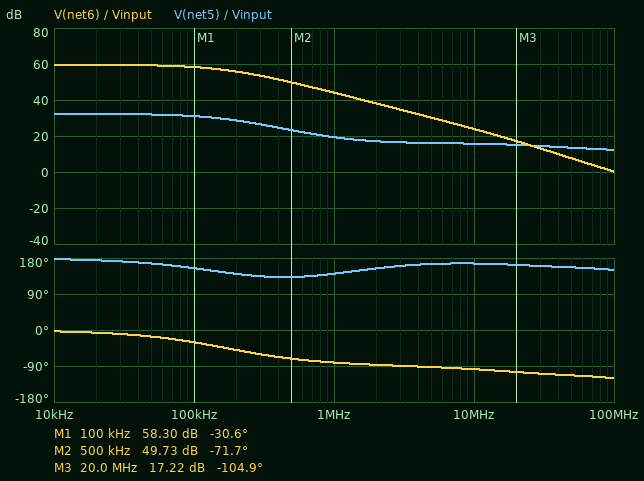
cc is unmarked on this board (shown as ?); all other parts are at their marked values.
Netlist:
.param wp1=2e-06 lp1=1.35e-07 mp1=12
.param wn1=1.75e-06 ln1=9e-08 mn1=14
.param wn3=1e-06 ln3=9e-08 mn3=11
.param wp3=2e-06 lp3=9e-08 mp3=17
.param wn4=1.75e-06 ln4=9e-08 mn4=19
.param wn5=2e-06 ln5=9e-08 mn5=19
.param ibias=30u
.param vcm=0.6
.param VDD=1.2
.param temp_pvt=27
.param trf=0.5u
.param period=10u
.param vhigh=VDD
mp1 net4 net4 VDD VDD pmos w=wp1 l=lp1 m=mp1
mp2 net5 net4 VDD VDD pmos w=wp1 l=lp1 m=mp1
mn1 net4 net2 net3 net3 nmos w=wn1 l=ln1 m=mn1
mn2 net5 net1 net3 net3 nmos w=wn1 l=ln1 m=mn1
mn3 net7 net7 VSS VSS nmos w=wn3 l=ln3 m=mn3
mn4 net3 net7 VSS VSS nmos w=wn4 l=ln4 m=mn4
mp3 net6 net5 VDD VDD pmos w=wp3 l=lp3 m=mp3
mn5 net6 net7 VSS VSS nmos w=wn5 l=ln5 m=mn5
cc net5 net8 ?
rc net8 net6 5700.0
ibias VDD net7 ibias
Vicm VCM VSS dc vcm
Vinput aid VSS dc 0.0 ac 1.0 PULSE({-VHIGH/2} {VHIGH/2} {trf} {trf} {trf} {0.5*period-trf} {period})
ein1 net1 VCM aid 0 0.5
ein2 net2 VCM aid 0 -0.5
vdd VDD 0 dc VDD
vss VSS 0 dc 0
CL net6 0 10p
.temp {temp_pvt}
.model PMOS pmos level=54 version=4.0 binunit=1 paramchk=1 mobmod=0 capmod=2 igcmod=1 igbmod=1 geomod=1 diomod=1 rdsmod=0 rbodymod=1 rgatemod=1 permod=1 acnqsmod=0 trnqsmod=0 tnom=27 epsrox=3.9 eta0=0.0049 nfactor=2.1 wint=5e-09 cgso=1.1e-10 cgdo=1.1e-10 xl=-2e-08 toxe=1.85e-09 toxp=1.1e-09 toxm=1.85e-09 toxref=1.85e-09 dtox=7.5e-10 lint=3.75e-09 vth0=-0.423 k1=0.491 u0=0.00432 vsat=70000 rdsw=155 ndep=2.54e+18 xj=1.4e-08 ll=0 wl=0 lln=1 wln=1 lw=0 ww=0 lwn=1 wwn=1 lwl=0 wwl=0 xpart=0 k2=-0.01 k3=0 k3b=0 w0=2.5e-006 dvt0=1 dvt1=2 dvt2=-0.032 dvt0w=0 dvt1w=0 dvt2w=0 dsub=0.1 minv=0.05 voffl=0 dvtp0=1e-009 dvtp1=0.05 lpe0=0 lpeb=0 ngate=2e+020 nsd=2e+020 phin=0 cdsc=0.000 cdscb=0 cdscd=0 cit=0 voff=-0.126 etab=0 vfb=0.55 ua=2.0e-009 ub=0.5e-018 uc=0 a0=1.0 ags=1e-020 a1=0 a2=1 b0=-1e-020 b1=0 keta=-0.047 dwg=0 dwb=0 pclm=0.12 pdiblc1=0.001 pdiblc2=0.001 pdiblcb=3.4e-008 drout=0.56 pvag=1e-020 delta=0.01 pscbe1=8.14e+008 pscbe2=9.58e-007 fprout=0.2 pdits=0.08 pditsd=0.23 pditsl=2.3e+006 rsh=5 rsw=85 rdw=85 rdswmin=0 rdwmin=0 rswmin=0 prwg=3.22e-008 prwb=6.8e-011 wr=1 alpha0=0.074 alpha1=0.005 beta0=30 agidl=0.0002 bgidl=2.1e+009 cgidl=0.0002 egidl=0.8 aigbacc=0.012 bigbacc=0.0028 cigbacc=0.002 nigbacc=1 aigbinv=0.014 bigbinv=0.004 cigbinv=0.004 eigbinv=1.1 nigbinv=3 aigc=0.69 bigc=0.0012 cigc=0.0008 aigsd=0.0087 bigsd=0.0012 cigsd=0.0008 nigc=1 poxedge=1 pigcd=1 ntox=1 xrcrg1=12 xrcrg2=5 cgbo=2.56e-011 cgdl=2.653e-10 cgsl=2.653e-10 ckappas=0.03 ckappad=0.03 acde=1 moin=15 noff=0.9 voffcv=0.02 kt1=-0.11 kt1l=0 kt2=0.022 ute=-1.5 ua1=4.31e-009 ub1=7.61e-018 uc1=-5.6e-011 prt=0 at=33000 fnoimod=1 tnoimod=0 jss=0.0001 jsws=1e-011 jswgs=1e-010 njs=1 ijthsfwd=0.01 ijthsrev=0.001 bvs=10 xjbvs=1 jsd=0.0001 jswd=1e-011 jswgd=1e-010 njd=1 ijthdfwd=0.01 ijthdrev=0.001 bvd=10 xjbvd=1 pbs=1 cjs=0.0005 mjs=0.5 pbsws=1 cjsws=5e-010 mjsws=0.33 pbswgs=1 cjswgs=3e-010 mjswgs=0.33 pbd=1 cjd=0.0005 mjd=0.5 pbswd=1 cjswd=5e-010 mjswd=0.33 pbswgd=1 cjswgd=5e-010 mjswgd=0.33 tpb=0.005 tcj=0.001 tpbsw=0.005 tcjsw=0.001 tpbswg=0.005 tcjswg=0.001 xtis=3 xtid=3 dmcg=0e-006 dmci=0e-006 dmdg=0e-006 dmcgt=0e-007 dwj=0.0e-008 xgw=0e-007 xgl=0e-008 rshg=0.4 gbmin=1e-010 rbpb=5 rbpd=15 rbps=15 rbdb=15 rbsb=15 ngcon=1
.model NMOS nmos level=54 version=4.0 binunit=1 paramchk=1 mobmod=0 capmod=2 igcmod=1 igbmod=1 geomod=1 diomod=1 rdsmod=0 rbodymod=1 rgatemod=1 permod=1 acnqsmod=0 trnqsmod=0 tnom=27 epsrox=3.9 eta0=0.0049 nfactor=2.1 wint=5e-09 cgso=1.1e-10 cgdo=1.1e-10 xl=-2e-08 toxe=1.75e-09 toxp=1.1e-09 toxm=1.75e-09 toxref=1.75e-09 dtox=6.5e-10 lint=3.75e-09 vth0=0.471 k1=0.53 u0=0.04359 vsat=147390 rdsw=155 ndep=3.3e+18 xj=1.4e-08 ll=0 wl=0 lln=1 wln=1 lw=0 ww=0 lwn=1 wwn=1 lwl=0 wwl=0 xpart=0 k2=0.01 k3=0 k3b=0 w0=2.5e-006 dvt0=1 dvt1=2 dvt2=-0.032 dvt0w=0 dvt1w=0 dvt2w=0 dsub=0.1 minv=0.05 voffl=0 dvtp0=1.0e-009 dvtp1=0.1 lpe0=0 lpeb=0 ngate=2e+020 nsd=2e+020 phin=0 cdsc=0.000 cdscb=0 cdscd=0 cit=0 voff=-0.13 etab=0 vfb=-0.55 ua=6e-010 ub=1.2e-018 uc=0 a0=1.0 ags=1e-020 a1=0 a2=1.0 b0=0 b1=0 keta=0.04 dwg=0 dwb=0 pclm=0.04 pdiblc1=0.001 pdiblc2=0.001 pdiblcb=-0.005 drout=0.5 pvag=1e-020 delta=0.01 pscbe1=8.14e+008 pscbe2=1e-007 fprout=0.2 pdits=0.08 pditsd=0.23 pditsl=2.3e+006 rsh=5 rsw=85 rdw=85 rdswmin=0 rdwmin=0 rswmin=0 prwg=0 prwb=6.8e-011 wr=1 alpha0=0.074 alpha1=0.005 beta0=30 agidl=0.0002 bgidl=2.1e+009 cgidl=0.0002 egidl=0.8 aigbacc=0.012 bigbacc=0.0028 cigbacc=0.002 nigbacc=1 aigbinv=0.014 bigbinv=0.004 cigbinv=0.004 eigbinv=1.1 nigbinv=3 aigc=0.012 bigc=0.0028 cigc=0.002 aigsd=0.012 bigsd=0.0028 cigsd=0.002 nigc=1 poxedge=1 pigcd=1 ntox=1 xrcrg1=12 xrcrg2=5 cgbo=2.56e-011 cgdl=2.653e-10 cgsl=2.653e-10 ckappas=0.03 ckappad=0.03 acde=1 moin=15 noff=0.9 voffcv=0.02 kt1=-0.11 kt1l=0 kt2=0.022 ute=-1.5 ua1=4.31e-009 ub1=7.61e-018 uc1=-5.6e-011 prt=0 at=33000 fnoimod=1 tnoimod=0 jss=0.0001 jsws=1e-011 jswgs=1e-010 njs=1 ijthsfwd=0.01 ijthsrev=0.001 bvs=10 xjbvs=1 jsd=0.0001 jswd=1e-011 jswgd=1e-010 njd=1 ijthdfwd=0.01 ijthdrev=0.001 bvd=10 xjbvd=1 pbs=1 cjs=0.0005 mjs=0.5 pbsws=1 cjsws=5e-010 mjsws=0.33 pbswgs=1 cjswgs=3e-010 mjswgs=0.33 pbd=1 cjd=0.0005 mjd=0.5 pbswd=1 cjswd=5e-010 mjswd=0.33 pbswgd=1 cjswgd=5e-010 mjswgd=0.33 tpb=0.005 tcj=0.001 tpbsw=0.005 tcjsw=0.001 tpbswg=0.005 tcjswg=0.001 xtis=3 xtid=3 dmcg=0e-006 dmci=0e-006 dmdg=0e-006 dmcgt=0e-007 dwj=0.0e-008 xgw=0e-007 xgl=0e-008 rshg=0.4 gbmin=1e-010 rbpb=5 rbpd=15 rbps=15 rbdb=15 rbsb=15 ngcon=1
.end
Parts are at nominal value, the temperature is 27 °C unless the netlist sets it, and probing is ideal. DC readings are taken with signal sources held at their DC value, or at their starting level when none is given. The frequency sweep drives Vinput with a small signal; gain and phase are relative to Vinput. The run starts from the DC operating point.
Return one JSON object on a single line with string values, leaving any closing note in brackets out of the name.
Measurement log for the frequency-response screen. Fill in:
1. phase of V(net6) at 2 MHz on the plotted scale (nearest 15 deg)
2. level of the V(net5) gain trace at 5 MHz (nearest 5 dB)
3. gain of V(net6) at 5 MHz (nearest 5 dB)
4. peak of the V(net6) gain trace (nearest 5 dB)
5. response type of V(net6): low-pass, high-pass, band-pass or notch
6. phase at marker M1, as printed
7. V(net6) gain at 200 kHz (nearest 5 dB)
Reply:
{"phase of V(net6) at 2 MHz on the plotted scale": "-90 deg", "level of the V(net5) gain trace at 5 MHz": "15 dB", "gain of V(net6) at 5 MHz": "30 dB", "peak of the V(net6) gain trace": "60 dB", "response type of V(net6): low-pass, high-pass, band-pass or notch": "low-pass", "phase at marker M1, as printed": "-30.6 deg", "V(net6) gain at 200 kHz": "55 dB"}
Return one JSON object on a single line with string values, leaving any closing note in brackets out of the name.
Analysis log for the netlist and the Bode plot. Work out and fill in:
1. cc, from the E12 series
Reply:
{"cc, from the E12 series": "680 fF"}
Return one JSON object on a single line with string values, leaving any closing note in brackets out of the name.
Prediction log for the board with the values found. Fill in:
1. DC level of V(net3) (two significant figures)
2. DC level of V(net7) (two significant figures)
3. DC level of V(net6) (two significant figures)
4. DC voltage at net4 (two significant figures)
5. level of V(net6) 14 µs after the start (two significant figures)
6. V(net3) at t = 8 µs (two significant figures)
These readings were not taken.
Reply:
{"DC level of V(net3)": "240 mV", "DC level of V(net7)": "380 mV", "DC level of V(net6)": "710 mV", "DC voltage at net4": "710 mV", "level of V(net6) 14 µs after the start": "1.2 V", "V(net3) at t = 8 µs": "500 mV"}
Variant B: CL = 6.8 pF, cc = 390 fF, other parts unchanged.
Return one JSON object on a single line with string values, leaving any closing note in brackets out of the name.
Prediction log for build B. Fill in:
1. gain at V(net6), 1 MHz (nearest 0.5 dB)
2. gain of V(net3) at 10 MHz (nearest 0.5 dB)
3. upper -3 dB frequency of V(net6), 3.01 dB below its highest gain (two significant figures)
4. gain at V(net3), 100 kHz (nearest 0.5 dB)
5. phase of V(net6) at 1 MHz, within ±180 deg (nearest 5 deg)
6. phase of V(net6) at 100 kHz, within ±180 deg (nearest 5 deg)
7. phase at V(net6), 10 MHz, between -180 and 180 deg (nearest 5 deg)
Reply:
{"gain at V(net6), 1 MHz": "48.5 dB", "gain of V(net3) at 10 MHz": "-21.5 dB", "upper -3 dB frequency of V(net6), 3.01 dB below its highest gain": "280 kHz", "gain at V(net3), 100 kHz": "-9.5 dB", "phase of V(net6) at 1 MHz, within ±180 deg": "-75 deg", "phase of V(net6) at 100 kHz, within ±180 deg": "-20 deg", "phase at V(net6), 10 MHz, between -180 and 180 deg": "-95 deg"}
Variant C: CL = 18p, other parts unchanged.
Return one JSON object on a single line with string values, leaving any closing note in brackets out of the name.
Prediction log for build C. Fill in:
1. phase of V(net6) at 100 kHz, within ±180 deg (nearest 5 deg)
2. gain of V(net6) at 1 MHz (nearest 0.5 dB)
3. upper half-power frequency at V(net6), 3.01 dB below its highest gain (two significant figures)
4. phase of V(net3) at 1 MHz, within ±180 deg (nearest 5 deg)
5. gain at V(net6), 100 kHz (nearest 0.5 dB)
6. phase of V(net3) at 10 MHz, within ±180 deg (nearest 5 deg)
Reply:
{"phase of V(net6) at 100 kHz, within ±180 deg": "-35 deg", "gain of V(net6) at 1 MHz": "43.0 dB", "upper half-power frequency at V(net6), 3.01 dB below its highest gain": "150 kHz", "phase of V(net3) at 1 MHz, within ±180 deg": "155 deg", "gain at V(net6), 100 kHz": "58.0 dB", "phase of V(net3) at 10 MHz, within ±180 deg": "160 deg"}
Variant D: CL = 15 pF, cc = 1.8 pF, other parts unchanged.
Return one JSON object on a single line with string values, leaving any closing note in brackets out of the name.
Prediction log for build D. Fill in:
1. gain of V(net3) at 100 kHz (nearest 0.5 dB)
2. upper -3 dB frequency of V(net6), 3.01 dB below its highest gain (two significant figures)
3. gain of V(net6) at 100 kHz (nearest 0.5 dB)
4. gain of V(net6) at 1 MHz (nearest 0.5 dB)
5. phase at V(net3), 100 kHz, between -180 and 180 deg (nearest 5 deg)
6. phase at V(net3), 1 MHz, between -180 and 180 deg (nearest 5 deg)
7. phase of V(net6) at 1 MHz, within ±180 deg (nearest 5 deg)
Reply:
{"gain of V(net3) at 100 kHz": "-14.0 dB", "upper -3 dB frequency of V(net6), 3.01 dB below its highest gain": "69 kHz", "gain of V(net6) at 100 kHz": "54.5 dB", "gain of V(net6) at 1 MHz": "36.5 dB", "phase at V(net3), 100 kHz, between -180 and 180 deg": "135 deg", "phase at V(net3), 1 MHz, between -180 and 180 deg": "150 deg", "phase of V(net6) at 1 MHz, within ±180 deg": "-85 deg"}
